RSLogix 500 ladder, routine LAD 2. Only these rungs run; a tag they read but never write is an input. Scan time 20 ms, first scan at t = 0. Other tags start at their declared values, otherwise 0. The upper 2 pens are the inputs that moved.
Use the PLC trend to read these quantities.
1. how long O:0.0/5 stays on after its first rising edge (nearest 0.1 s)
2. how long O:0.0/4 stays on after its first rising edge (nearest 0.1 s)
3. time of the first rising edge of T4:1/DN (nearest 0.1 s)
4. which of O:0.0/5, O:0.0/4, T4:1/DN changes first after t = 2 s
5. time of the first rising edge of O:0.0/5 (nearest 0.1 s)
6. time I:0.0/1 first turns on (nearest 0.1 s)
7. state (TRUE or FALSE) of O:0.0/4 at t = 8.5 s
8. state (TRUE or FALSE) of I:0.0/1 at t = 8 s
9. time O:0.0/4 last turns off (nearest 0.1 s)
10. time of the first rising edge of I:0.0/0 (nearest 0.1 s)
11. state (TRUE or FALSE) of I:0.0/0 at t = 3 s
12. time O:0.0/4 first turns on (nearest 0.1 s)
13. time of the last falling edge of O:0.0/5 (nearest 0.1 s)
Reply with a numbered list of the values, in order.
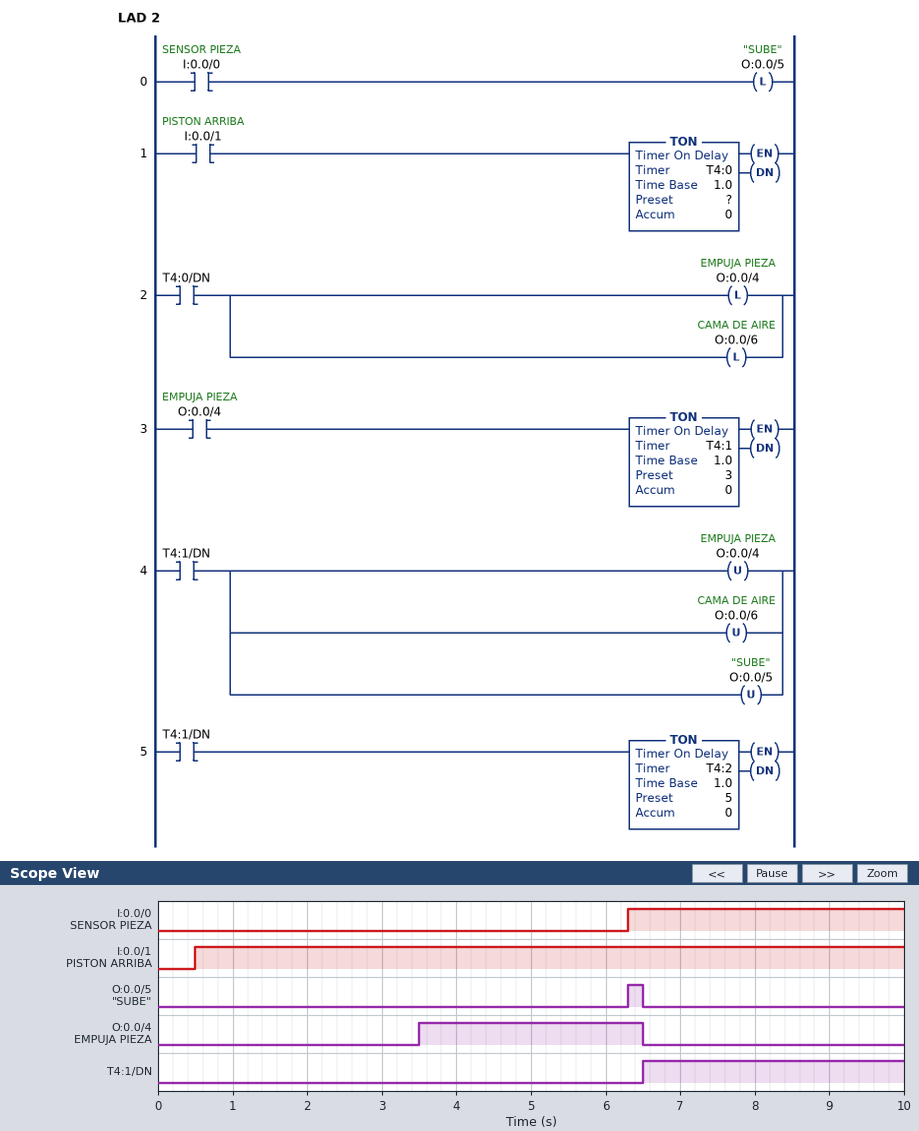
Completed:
1. 0.2 s
2. 3.0 s
3. 6.5 s
4. O:0.0/4
5. 6.3 s
6. 0.5 s
7. FALSE
8. TRUE
9. 6.5 s
10. 6.3 s
11. FALSE
12. 3.5 s
13. 6.5 s
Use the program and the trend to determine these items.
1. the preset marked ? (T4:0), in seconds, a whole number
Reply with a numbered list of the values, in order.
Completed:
1. 3 s
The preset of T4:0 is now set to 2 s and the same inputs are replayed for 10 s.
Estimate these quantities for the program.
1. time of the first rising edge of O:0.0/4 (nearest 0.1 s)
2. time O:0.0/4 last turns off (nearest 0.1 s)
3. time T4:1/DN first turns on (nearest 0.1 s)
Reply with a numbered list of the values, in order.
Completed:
1. 2.5 s
2. 5.5 s
3. 5.5 s
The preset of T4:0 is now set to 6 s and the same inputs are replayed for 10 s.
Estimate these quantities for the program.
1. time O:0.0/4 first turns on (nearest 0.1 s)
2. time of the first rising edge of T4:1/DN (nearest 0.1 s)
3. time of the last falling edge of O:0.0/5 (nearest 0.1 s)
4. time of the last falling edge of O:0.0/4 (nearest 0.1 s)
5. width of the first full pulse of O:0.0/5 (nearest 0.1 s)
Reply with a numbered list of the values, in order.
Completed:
1. 6.5 s
2. 9.5 s
3. 9.5 s
4. 9.5 s
5. 3.2 s
